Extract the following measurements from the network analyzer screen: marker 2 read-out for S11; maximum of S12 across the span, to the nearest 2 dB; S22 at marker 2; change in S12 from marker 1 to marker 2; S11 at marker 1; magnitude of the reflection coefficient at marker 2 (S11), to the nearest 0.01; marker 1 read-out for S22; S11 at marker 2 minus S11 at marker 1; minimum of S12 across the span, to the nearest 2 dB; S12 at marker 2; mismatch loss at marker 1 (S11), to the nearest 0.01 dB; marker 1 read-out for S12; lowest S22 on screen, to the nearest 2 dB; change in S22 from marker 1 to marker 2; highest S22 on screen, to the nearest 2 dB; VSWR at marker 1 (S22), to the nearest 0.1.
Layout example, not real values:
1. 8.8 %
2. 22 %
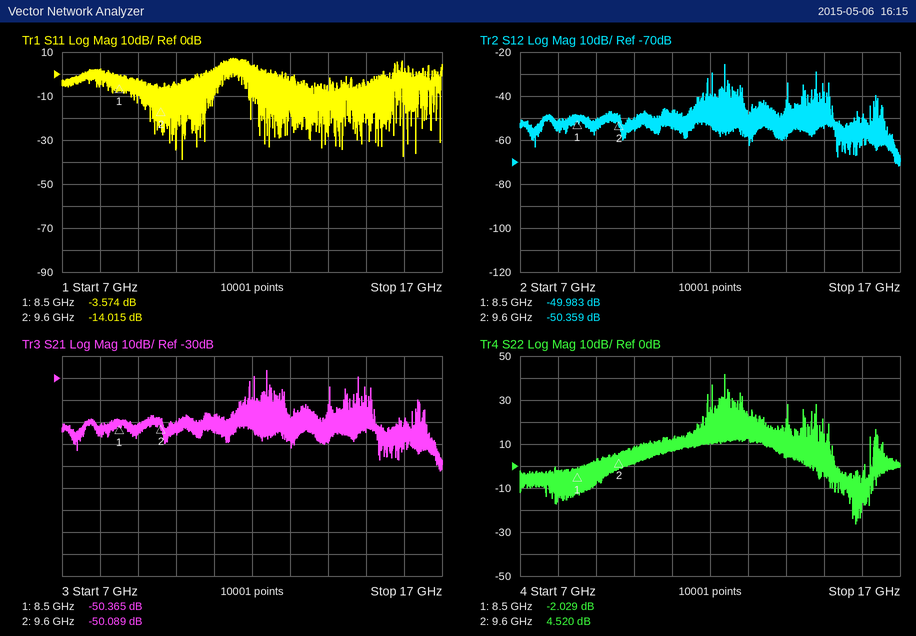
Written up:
1. -14.015 dB
2. -26 dB
3. 4.520 dB
4. -0.376 dB
5. -3.574 dB
6. 0.20
7. -2.029 dB
8. -10.441 dB
9. -72 dB
10. -50.359 dB
11. 2.51 dB
12. -49.983 dB
13. -26 dB
14. 6.549 dB
15. 42 dB
16. 8.6
